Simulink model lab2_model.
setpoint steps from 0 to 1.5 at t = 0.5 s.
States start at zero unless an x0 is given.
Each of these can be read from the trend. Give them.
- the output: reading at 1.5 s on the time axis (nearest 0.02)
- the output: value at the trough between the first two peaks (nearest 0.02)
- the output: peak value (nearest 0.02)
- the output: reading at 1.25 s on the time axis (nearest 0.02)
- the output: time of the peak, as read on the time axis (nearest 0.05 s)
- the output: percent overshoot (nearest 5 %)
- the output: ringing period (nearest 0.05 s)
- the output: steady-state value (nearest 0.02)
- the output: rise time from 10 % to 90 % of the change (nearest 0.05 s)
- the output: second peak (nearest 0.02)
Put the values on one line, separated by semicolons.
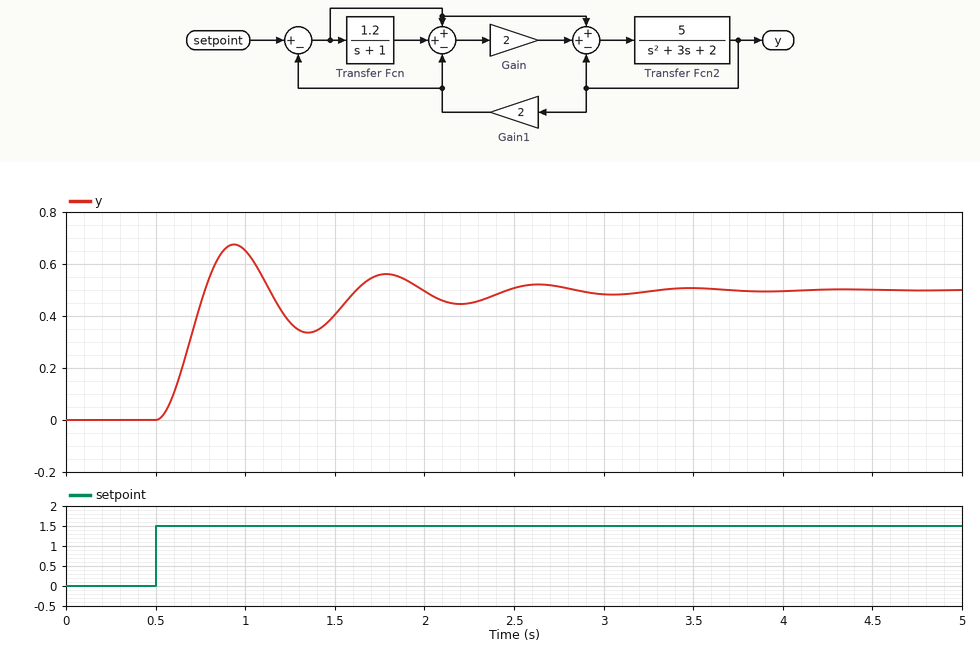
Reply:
0.40; 0.34; 0.68; 0.38; 0.95 s; 35 %; 0.85 s; 0.50; 0.20 s; 0.56
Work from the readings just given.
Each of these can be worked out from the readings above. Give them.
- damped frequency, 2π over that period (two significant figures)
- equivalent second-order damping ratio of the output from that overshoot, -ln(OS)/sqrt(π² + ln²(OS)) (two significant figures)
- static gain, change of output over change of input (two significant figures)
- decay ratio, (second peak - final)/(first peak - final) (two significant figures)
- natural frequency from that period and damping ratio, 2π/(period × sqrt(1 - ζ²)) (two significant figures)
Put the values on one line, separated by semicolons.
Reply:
7.4 rad/s; 0.32; 0.33; 0.33; 7.8 rad/s
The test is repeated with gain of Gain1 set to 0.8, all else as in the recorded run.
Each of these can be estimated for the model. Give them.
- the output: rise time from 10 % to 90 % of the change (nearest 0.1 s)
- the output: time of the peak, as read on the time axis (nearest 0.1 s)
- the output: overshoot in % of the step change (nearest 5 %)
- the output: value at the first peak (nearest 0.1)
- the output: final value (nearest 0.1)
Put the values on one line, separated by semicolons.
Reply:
0.3 s; 1.2 s; 25 %; 1.4; 1.1
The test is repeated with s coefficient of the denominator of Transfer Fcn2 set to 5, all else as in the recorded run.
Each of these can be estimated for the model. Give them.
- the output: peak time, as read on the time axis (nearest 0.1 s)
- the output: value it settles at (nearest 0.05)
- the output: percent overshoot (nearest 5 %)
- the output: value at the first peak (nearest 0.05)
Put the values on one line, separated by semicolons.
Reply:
1.0 s; 0.50; 20 %; 0.60
